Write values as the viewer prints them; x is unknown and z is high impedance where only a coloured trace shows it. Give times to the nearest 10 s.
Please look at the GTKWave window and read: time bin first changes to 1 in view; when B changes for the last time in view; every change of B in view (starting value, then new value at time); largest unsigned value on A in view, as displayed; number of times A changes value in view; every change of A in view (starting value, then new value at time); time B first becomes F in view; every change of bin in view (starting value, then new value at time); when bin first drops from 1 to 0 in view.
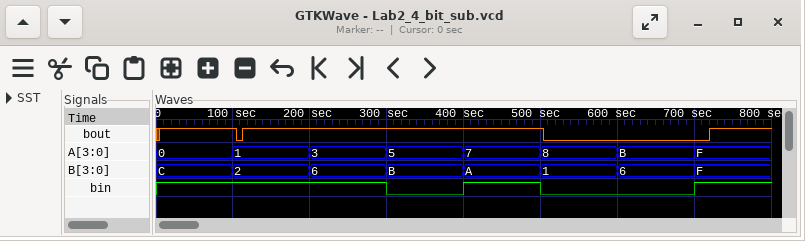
400 s
700 s
C, 2 at 100 s, 6 at 200 s, B at 300 s, A at 400 s, 1 at 500 s, 6 at 600 s, F at 700 s
F
7
0, 1 at 100 s, 3 at 200 s, 5 at 300 s, 7 at 400 s, 8 at 500 s, B at 600 s, F at 700 s
700 s
1, 0 at 300 s, 1 at 400 s, 0 at 500 s, 1 at 700 s
300 s
